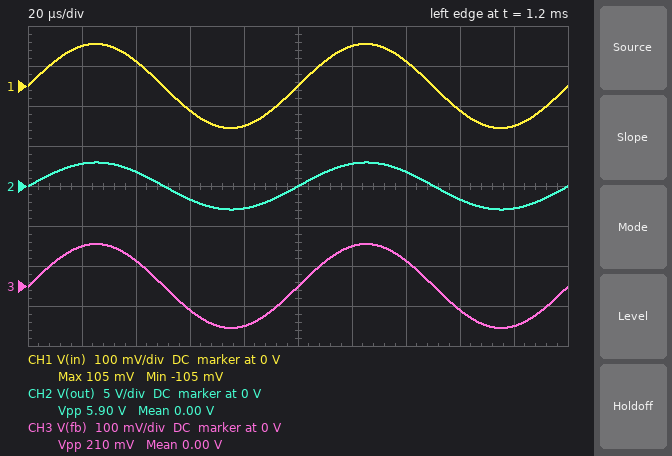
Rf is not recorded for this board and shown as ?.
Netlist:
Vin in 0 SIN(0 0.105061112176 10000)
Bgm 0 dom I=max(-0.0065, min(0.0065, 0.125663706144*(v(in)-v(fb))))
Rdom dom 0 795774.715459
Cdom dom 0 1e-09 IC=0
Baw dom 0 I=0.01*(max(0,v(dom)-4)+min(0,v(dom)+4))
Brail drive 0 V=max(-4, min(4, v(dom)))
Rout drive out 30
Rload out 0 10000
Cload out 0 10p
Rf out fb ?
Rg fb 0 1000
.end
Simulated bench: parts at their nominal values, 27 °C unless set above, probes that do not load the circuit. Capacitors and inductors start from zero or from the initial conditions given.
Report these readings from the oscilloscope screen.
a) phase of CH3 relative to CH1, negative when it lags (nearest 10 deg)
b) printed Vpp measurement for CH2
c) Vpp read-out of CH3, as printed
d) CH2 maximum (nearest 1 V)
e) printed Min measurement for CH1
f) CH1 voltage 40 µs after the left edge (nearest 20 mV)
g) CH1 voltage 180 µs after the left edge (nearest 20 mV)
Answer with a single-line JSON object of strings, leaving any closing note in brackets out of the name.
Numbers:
{"phase of CH3 relative to CH1, negative when it lags": "0 deg", "printed Vpp measurement for CH2": "5.90 V", "Vpp read-out of CH3, as printed": "210 mV", "CH2 maximum": "3 V", "printed Min measurement for CH1": "-105 mV", "CH1 voltage 40 µs after the left edge": "60 mV", "CH1 voltage 180 µs after the left edge": "-100 mV"}
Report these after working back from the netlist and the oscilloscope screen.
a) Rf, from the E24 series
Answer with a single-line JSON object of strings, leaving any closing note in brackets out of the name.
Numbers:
{"Rf, from the E24 series": "27 kΩ"}
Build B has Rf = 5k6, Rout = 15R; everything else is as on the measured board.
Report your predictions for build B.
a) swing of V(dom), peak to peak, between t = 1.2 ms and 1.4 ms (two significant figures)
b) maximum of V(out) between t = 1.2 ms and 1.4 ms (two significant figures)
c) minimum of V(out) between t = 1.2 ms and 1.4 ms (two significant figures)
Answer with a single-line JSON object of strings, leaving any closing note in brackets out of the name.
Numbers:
{"swing of V(dom), peak to peak, between t = 1.2 ms and 1.4 ms": "1.4 V", "maximum of V(out) between t = 1.2 ms and 1.4 ms": "690 mV", "minimum of V(out) between t = 1.2 ms and 1.4 ms": "-690 mV"}
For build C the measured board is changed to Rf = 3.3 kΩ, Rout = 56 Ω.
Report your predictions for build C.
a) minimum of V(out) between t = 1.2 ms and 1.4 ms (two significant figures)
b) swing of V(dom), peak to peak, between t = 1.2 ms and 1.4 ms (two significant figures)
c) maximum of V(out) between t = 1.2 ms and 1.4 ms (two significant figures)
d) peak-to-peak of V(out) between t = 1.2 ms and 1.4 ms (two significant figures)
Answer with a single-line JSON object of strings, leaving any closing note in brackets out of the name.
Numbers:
{"minimum of V(out) between t = 1.2 ms and 1.4 ms": "-450 mV", "swing of V(dom), peak to peak, between t = 1.2 ms and 1.4 ms": "920 mV", "maximum of V(out) between t = 1.2 ms and 1.4 ms": "450 mV", "peak-to-peak of V(out) between t = 1.2 ms and 1.4 ms": "900 mV"}
